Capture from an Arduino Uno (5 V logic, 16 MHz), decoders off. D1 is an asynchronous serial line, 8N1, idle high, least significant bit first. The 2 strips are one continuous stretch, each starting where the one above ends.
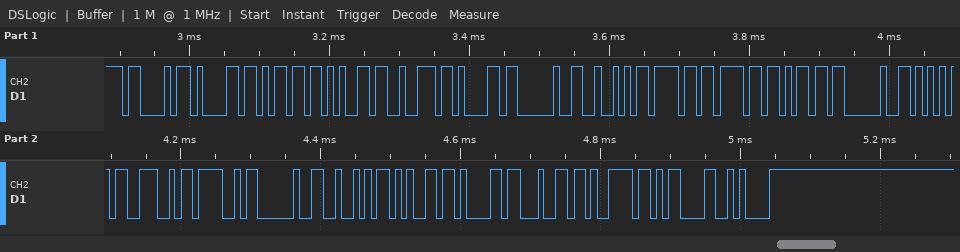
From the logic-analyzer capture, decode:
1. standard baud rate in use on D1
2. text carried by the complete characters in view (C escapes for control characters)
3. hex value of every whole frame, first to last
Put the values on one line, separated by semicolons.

115200 baud; "Camera Room UNO Ready\r\n"; 43 61 6D 65 72 61 20 52 6F 6F 6D 20 55 4E 4F 20 52 65 61 64 79 0D 0A
